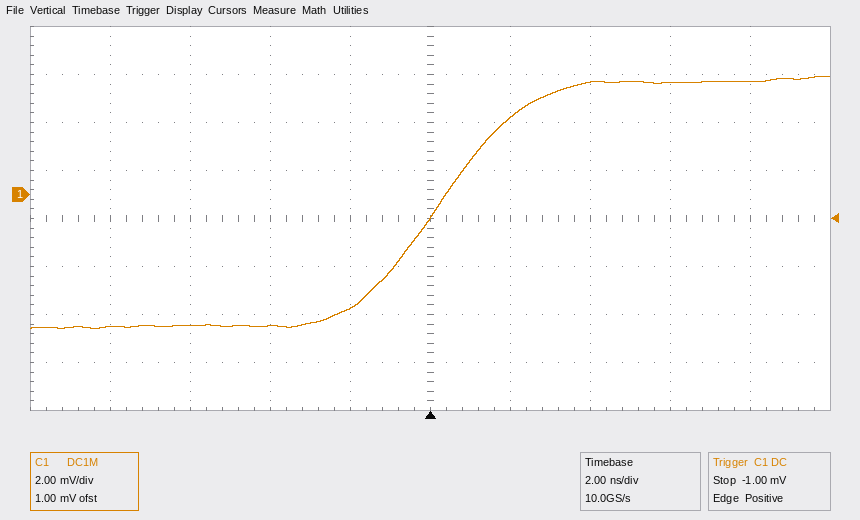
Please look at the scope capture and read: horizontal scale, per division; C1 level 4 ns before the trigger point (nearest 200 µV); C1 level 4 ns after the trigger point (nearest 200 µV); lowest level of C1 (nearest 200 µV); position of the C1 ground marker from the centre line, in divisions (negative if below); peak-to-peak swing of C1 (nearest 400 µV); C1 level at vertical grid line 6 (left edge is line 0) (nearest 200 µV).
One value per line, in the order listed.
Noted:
2 ns
-5.4 mV
4.6 mV
-5.6 mV
+0.5 div
10.4 mV
3.2 mV
